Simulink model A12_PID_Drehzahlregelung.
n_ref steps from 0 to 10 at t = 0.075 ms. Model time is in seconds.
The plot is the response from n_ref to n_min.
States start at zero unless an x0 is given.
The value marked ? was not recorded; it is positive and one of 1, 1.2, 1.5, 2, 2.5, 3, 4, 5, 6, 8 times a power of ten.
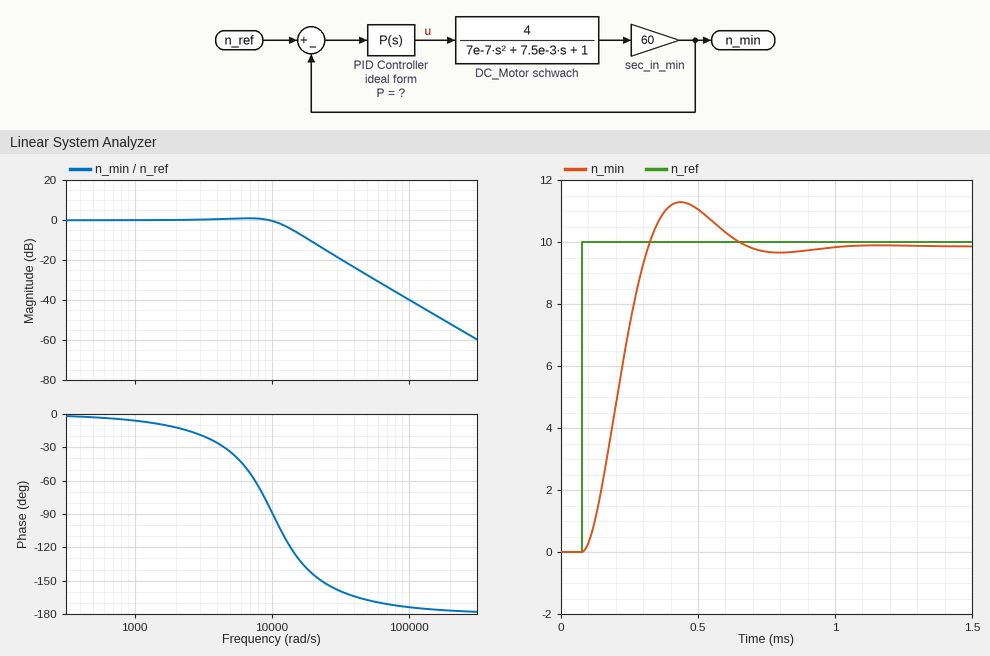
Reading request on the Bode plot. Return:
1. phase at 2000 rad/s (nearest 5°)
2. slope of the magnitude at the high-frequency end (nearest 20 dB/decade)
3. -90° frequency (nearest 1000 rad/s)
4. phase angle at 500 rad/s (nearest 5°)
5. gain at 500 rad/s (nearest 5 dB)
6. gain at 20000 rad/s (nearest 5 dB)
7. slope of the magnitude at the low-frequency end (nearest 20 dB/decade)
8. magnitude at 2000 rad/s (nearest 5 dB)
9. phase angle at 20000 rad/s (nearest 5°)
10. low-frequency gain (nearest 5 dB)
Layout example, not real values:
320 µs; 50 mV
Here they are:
-10°; -40 dB/decade; 10000 rad/s; -5°; 0 dB; -10 dB; 0 dB/decade; 0 dB; -145°; 0 dB
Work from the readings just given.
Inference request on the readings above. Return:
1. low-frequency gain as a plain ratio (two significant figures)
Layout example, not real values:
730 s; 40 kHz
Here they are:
1.0
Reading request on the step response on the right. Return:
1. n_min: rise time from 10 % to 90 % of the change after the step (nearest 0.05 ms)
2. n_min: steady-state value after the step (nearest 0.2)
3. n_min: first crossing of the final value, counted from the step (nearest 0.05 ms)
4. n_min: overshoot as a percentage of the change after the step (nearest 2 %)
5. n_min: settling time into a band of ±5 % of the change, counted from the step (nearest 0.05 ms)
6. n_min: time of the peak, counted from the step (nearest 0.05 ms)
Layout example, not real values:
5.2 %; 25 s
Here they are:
0.15 ms; 9.8; 0.25 ms; 14 %; 0.50 ms; 0.35 ms
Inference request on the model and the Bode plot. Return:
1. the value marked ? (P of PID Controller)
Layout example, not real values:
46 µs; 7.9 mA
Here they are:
0.3
